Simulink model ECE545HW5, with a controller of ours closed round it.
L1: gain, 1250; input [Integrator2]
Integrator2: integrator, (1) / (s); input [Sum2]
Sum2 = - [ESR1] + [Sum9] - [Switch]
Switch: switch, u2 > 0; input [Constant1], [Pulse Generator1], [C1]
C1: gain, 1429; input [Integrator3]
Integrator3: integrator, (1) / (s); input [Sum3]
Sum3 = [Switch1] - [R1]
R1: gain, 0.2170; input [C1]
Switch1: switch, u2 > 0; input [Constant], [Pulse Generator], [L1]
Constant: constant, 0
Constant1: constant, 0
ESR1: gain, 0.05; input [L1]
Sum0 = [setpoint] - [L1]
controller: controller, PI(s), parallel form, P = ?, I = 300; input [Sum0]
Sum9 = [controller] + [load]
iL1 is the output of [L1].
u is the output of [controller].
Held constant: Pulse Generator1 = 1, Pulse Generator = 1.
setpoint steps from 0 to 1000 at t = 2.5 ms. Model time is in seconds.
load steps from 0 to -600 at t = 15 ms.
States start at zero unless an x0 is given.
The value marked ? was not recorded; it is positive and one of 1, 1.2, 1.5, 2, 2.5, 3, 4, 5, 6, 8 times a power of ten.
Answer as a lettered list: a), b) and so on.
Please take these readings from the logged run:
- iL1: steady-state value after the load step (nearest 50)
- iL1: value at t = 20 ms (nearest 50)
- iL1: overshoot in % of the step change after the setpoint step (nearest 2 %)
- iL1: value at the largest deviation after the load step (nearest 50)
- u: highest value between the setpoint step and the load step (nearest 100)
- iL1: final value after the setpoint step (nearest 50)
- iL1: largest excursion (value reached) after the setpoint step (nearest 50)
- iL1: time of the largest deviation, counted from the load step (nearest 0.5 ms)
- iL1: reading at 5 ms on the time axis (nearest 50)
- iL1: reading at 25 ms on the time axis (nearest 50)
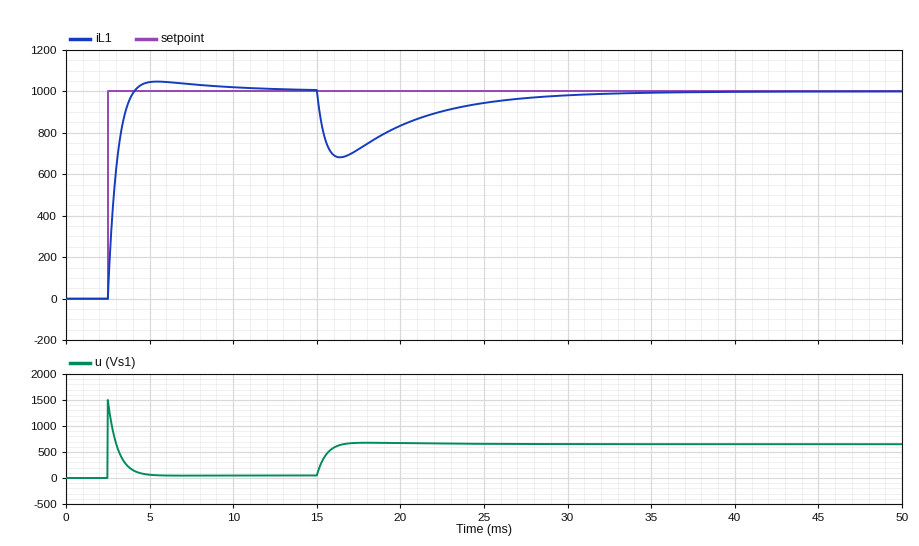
a) 1000
b) 850
c) 4 %
d) 700
e) 1500
f) 1000
g) 1050
h) 1.5 ms
i) 1050
j) 950
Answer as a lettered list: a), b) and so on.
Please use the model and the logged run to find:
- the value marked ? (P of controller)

a) 1.5
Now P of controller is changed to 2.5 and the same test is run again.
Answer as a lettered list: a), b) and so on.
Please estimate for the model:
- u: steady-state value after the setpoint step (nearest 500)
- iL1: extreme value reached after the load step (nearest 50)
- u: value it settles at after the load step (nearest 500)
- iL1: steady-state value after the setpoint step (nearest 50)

a) 0
b) 800
c) 500
d) 1000
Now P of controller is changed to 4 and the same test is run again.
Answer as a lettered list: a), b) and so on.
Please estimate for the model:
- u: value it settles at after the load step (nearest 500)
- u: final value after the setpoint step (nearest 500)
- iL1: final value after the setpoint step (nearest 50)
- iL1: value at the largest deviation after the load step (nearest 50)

a) 500
b) 0
c) 1000
d) 850
